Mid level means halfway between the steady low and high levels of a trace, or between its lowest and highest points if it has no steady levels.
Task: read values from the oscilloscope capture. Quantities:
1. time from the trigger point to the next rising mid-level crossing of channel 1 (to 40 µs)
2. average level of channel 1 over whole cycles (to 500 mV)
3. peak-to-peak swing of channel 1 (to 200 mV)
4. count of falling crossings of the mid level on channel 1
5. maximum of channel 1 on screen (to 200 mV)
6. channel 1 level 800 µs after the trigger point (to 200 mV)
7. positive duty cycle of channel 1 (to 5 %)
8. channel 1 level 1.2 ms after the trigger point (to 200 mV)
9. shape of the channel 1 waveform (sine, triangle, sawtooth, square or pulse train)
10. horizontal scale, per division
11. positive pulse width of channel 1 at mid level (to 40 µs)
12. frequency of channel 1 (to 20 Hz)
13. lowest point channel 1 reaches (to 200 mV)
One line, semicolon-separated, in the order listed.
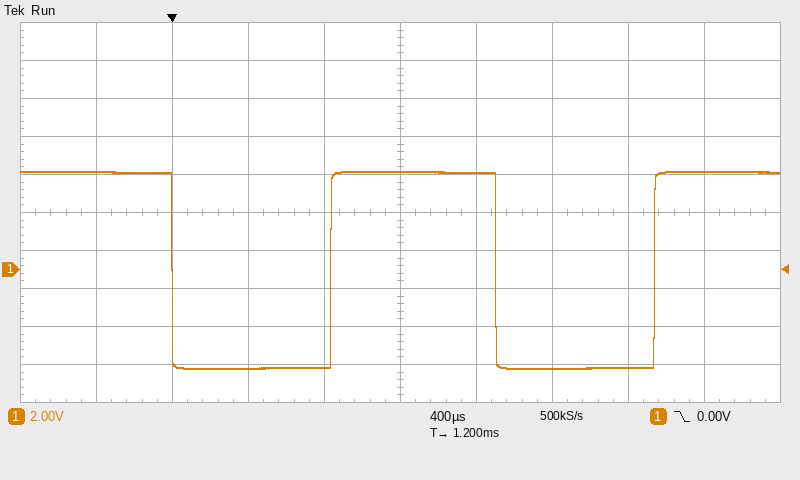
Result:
840 µs; 0.0 V; 10.4 V; 2; 5.2 V; -5.2 V; 50 %; 5.2 V; square; 400 µs; 880 µs; 580 Hz; -5.2 V
